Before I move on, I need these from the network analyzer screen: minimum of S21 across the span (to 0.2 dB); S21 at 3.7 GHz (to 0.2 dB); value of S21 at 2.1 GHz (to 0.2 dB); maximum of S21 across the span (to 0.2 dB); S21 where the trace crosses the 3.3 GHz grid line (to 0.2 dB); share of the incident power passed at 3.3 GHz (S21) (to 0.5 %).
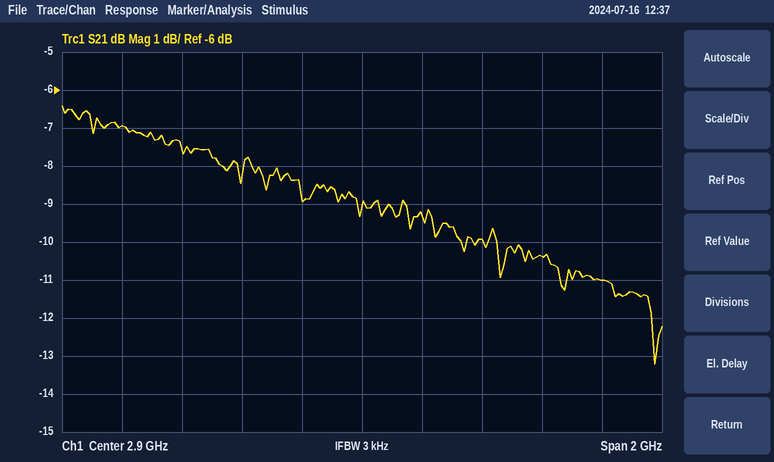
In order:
-13.2 dB
-11.0 dB
-7.0 dB
-6.4 dB
-10.0 dB
10.0 %
